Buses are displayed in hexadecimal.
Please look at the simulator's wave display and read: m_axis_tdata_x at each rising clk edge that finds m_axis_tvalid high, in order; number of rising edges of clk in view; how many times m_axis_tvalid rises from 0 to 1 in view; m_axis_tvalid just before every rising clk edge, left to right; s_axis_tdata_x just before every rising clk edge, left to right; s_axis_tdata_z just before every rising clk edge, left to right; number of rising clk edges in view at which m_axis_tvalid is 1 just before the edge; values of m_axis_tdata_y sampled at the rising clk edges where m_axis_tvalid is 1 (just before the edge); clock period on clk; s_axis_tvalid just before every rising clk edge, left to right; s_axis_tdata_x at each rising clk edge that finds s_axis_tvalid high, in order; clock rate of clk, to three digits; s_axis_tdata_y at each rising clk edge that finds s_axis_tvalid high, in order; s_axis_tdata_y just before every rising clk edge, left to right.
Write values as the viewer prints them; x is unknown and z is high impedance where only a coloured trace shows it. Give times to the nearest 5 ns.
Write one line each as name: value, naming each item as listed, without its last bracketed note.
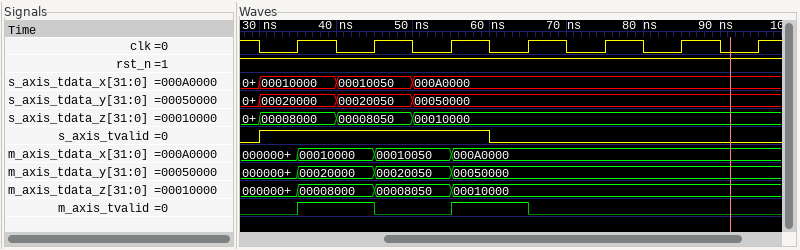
m_axis_tdata_x at each rising clk edge that finds m_axis_tvalid high, in order: 00010000, 000A0000
number of rising edges of clk in view: 7
how many times m_axis_tvalid rises from 0 to 1 in view: 2
m_axis_tvalid just before every rising clk edge, left to right: 0 1 0 1 0 0 0
s_axis_tdata_x just before every rising clk edge, left to right: 00010000, 00010050, 000A0000, 000A0000, 000A0000, 000A0000, 000A0000
s_axis_tdata_z just before every rising clk edge, left to right: 00008000, 00008050, 00010000, 00010000, 00010000, 00010000, 00010000
number of rising clk edges in view at which m_axis_tvalid is 1 just before the edge: 2
values of m_axis_tdata_y sampled at the rising clk edges where m_axis_tvalid is 1: 00020000, 00050000
clock period on clk: 10 ns
s_axis_tvalid just before every rising clk edge, left to right: 1 1 1 0 0 0 0
s_axis_tdata_x at each rising clk edge that finds s_axis_tvalid high, in order: 00010000, 00010050, 000A0000
clock rate of clk, to three digits: 100 MHz
s_axis_tdata_y at each rising clk edge that finds s_axis_tvalid high, in order: 00020000, 00020050, 00050000
s_axis_tdata_y just before every rising clk edge, left to right: 00020000, 00020050, 00050000, 00050000, 00050000, 00050000, 00050000
